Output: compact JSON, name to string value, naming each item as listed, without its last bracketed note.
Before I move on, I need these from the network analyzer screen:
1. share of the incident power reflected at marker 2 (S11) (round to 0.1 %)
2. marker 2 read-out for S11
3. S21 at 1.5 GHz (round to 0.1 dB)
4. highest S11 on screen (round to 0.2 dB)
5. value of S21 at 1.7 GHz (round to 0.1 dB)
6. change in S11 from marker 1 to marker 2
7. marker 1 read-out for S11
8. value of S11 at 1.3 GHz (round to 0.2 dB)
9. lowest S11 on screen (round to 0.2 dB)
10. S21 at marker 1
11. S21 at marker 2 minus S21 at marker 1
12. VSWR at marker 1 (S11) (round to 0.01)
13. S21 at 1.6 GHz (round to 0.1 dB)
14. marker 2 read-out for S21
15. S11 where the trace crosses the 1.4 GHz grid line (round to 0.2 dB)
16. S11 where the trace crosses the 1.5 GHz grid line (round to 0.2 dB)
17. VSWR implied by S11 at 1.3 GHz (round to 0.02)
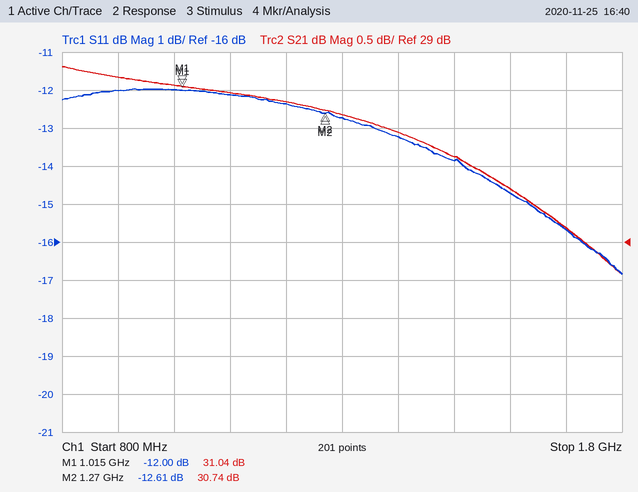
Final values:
{"share of the incident power reflected at marker 2 (S11)": "5.5 %", "marker 2 read-out for S11": "-12.61 dB", "S21 at 1.5 GHz": "30.1 dB", "highest S11 on screen": "-12.0 dB", "value of S21 at 1.7 GHz": "29.2 dB", "change in S11 from marker 1 to marker 2": "-0.61 dB", "marker 1 read-out for S11": "-12.00 dB", "value of S11 at 1.3 GHz": "-12.8 dB", "lowest S11 on screen": "-16.8 dB", "S21 at marker 1": "31.04 dB", "S21 at marker 2 minus S21 at marker 1": "-0.30 dB", "VSWR at marker 1 (S11)": "1.67", "S21 at 1.6 GHz": "29.7 dB", "marker 2 read-out for S21": "30.74 dB", "S11 where the trace crosses the 1.4 GHz grid line": "-13.2 dB", "S11 where the trace crosses the 1.5 GHz grid line": "-13.8 dB", "VSWR implied by S11 at 1.3 GHz": "1.60"}
